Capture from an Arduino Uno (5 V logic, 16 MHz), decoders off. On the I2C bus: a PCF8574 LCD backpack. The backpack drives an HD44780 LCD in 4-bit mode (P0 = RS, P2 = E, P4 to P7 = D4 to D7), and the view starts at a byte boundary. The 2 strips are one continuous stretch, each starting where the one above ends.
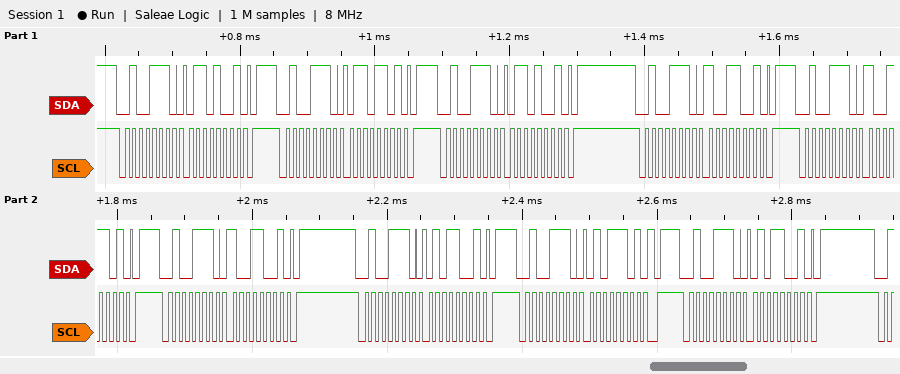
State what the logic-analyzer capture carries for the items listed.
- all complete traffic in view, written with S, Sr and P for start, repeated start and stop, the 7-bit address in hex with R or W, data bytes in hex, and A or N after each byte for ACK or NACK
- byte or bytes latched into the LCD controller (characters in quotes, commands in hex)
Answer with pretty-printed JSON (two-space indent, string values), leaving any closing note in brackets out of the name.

{
  "all complete traffic in view, written with S, Sr and P for start, repeated start and stop, the 7-bit address in hex with R or W, data bytes in hex, and A or N after each byte for ACK or NACK": "S 27W A 69 A P S 27W A 6D A P S 27W A 69 A P S 27W A 99 A P S 27W A 9D A P S 27W A 99 A P S 27W A 59 A P S 27W A 5D A P S 27W A 59 A P",
  "byte or bytes latched into the LCD controller": "'i'"
}
